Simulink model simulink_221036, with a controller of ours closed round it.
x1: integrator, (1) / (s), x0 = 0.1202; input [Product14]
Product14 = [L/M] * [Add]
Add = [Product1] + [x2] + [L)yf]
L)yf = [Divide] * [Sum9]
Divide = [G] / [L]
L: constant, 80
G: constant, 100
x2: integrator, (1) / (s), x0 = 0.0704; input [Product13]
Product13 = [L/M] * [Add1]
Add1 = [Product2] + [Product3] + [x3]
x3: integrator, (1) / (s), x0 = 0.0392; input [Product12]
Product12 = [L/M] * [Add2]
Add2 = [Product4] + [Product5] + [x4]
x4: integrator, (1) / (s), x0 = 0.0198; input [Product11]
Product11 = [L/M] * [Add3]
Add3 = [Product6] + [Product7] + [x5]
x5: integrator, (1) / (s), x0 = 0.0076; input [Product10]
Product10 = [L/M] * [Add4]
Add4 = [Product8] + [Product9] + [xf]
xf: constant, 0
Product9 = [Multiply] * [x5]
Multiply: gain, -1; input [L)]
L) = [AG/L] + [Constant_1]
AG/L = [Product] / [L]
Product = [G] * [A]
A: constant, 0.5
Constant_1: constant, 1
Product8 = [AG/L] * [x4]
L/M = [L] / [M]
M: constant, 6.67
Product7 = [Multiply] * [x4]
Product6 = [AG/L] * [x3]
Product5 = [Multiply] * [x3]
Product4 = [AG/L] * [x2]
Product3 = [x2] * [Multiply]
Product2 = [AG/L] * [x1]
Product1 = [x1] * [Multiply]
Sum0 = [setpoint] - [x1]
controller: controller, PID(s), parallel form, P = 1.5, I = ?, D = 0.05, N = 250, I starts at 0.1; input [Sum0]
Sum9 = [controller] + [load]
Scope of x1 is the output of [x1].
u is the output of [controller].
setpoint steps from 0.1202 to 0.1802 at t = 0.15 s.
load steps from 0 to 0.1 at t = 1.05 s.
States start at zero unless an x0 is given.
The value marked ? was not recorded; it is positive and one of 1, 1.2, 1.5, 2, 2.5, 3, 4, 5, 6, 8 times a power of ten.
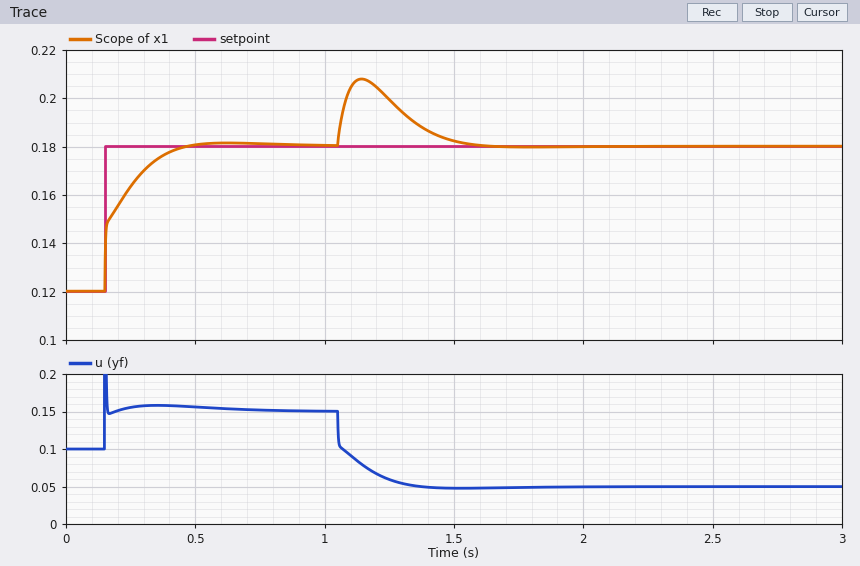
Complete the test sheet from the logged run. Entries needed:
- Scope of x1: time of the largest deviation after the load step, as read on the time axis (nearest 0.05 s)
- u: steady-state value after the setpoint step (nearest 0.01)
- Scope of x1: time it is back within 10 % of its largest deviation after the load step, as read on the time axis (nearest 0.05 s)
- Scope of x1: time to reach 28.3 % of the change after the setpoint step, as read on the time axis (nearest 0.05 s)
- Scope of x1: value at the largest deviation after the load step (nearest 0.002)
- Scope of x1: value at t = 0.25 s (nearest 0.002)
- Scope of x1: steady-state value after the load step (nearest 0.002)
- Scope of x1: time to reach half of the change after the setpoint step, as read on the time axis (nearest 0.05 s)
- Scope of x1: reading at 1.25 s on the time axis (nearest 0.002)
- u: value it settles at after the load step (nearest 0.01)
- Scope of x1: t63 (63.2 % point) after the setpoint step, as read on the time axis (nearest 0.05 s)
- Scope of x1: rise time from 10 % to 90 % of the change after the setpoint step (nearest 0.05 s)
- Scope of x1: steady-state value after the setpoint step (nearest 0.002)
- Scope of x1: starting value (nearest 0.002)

1.15 s
0.15
1.50 s
0.15 s
0.208
0.164
0.180
0.15 s
0.200
0.05
0.20 s
0.20 s
0.180
0.120
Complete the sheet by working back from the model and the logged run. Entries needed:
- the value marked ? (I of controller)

15
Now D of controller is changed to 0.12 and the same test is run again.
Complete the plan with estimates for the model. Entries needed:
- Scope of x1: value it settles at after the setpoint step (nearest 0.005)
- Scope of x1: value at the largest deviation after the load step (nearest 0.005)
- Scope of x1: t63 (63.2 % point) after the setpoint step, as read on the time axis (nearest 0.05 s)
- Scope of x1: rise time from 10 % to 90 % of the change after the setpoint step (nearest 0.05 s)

0.180
0.205
0.15 s
0.25 s
